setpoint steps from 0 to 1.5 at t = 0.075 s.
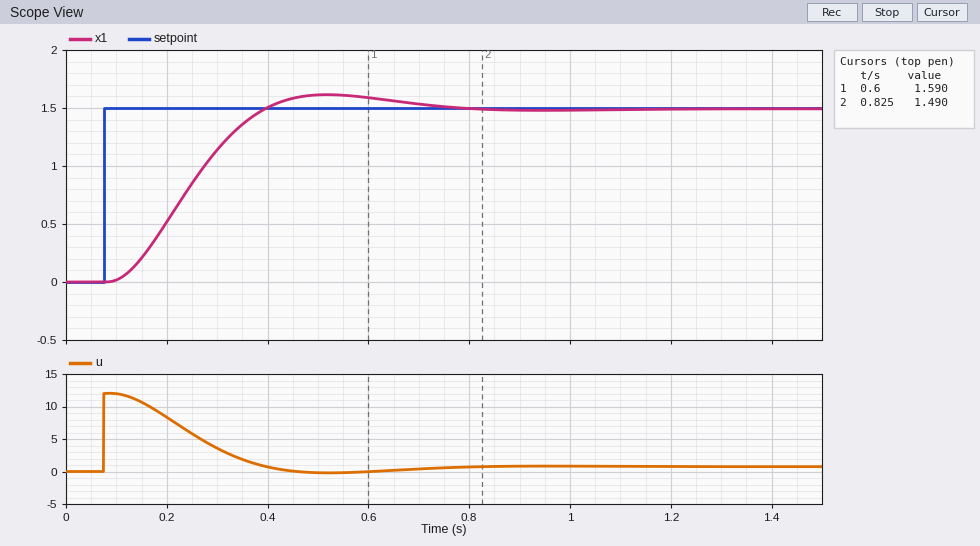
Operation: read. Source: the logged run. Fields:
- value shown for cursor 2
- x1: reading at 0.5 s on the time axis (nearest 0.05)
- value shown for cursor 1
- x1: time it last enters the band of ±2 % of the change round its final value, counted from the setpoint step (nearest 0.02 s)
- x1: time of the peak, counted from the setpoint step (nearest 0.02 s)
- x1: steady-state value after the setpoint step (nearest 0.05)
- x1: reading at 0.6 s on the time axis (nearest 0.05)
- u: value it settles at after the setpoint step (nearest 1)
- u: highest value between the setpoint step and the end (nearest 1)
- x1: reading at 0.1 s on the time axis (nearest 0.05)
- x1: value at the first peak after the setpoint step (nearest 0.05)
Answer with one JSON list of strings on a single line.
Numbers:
["1.490", "1.60", "1.590", "0.64 s", "0.44 s", "1.50", "1.60", "1", "12", "0.00", "1.60"]
